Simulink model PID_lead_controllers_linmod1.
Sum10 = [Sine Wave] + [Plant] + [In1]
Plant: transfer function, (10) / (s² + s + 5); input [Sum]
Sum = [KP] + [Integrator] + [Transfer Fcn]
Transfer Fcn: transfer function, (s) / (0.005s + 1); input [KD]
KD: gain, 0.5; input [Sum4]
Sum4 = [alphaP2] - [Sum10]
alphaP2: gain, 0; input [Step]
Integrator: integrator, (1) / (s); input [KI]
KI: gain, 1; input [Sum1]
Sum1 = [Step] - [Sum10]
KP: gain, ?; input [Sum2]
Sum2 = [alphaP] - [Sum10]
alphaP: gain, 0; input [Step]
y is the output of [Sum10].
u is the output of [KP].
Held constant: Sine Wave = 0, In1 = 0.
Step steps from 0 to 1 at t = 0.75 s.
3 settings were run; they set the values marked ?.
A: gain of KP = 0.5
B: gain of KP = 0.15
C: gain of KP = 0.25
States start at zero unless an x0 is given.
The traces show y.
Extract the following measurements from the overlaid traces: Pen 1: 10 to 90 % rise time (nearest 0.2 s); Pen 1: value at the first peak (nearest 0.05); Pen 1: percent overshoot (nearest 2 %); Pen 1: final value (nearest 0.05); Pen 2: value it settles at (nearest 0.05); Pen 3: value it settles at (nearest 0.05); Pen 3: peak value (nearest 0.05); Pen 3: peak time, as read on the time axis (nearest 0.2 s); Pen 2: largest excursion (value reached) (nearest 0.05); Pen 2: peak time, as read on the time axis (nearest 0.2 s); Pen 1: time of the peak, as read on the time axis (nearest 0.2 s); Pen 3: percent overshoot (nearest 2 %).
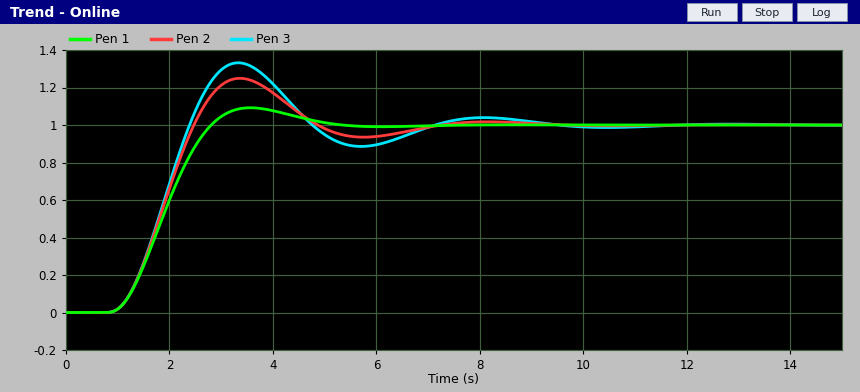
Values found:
1.2 s
1.10
10 %
1.00
1.00
1.00
1.35
3.4 s
1.25
3.4 s
3.6 s
34 %
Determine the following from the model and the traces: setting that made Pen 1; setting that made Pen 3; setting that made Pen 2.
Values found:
A
B
C
